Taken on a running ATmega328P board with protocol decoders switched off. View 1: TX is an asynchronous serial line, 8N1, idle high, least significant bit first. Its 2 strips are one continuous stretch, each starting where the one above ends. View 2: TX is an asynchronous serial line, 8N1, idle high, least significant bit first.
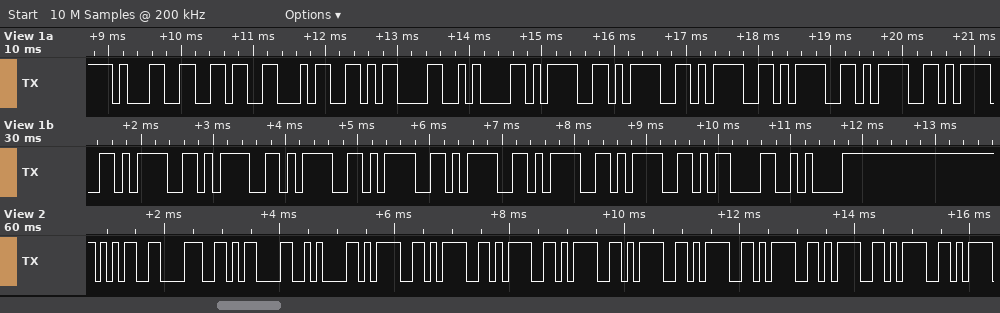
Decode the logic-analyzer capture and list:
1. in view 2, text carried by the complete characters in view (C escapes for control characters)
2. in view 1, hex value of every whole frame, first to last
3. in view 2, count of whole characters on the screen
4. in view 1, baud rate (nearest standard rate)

"58\r\n========="
31 36 34 0D 0A 3D 3D 3D 3D 3D 3D 3D 3D 3D 3D 3D 3D 3D 0D 0A
13
9600 baud
